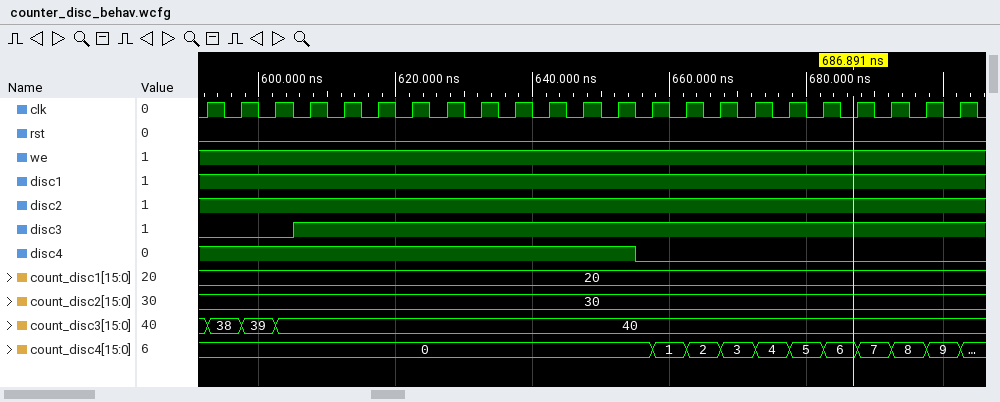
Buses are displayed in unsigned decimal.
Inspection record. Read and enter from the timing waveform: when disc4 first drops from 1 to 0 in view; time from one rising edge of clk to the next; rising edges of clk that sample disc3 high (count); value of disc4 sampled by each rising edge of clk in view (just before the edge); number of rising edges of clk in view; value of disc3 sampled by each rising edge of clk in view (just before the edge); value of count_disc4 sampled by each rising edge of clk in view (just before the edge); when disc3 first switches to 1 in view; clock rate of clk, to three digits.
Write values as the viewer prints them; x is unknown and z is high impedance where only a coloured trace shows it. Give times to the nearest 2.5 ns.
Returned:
655 ns
5 ns
20
1 1 1 1 1 1 1 1 1 1 1 1 1 0 0 0 0 0 0 0 0 0 0
23
0 0 0 1 1 1 1 1 1 1 1 1 1 1 1 1 1 1 1 1 1 1 1
0, 0, 0, 0, 0, 0, 0, 0, 0, 0, 0, 0, 0, 0, 1, 2, 3, 4, 5, 6, 7, 8, 9
605 ns
200 MHz
